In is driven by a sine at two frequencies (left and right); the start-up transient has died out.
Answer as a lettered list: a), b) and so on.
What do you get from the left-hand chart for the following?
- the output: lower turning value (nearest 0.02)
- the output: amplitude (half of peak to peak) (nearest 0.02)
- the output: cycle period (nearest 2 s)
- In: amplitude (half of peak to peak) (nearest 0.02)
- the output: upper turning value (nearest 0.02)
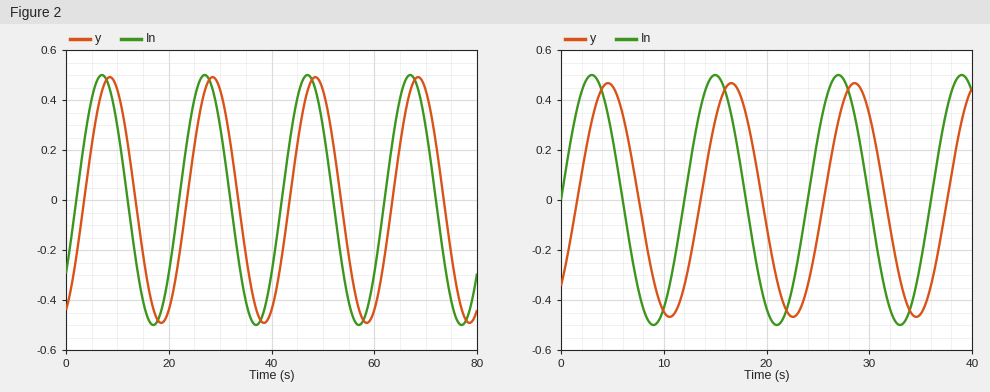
a) -0.50
b) 0.50
c) 20 s
d) 0.50
e) 0.50
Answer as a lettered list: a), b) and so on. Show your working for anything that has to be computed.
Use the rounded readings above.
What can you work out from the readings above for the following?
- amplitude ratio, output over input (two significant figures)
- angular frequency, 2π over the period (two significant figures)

a) 0.5 / 0.5 = 1.0
b) 2π / 20 = 0.31 rad/s
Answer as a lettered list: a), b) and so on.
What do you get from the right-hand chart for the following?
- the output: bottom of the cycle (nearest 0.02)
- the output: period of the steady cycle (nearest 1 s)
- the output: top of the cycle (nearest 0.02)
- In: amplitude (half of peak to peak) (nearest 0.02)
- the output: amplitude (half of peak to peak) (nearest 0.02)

a) -0.46
b) 12 s
c) 0.46
d) 0.50
e) 0.46
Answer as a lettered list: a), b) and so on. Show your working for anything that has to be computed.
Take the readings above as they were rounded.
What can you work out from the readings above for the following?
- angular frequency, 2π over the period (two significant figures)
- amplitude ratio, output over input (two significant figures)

a) 2π / 12 = 0.52 rad/s
b) 0.46 / 0.5 = 0.92
